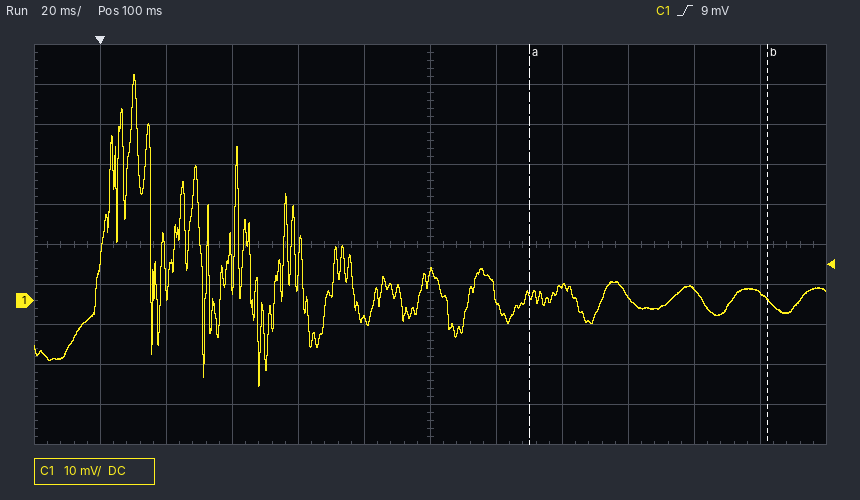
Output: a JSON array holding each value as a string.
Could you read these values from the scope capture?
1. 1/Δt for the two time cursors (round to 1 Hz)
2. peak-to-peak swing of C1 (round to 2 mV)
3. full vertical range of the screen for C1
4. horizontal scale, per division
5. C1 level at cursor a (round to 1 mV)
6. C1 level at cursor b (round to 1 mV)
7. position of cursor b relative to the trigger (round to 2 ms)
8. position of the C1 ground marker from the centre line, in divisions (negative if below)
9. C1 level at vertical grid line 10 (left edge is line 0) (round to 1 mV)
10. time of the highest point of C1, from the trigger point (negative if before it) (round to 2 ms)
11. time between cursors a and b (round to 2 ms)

["14 Hz", "78 mV", "100 mV", "20 ms", "1 mV", "0 mV", "+202 ms", "-1.4 div", "3 mV", "+10 ms", "72 ms"]
